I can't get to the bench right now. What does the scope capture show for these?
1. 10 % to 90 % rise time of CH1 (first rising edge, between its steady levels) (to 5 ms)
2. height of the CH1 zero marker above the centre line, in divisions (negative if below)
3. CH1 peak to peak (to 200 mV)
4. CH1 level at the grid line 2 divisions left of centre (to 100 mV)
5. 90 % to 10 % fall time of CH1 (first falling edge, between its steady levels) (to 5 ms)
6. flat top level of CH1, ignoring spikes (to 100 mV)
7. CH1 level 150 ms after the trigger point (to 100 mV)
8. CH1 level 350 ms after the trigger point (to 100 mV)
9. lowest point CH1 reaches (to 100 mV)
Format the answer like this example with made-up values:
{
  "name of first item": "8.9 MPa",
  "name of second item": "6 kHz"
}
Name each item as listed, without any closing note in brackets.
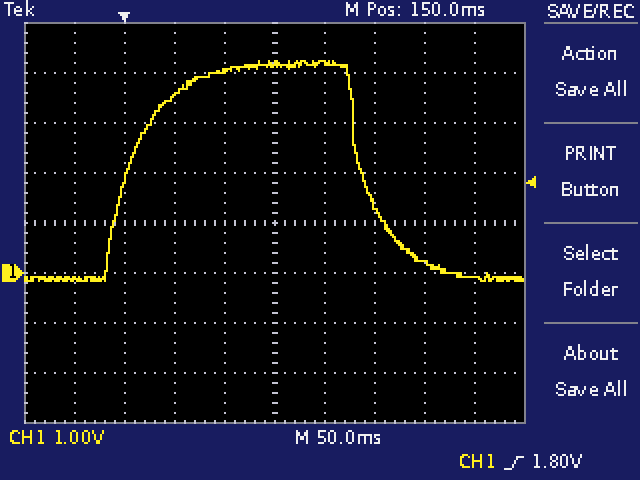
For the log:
{
  "10 % to 90 % rise time of CH1 (first rising edge, between its steady levels)": "80 ms",
  "height of the CH1 zero marker above the centre line, in divisions": "-1.0 div",
  "CH1 peak to peak": "4.4 V",
  "CH1 level at the grid line 2 divisions left of centre": "3.5 V",
  "90 % to 10 % fall time of CH1 (first falling edge, between its steady levels)": "65 ms",
  "flat top level of CH1, ignoring spikes": "4.2 V",
  "CH1 level 150 ms after the trigger point": "4.2 V",
  "CH1 level 350 ms after the trigger point": "-100 mV",
  "lowest point CH1 reaches": "-200 mV"
}
